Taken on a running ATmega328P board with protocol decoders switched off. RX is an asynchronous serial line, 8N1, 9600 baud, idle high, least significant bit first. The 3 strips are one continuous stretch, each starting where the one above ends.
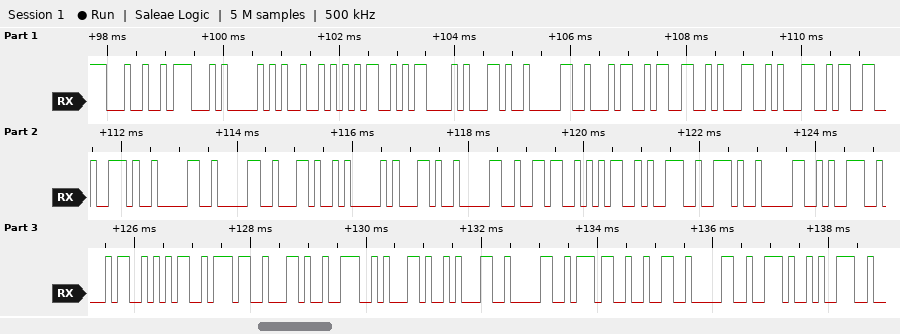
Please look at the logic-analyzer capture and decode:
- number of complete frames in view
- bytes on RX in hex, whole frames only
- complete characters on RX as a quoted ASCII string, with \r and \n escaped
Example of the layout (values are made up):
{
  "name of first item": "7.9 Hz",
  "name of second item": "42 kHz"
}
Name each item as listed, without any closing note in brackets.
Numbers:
{
  "number of complete frames in view": "39",
  "bytes on RX in hex, whole frames only": "0x24 0x47 0x50 0x52 0x4D 0x43 0x2C 0x30 0x34 0x33 0x31 0x31 0x33 0x2E 0x30 0x30 0x2C 0x41 0x2C 0x30 0x36 0x35 0x39 0x2E 0x30 0x39 0x34 0x35 0x37 0x2C 0x4E 0x2C 0x31 0x30 0x37 0x32 0x30 0x2E 0x39",
  "complete characters on RX as a quoted ASCII string, with \\r and \\n escaped": "\"$GPRMC,043113.00,A,0659.09457,N,10720.9\""
}
